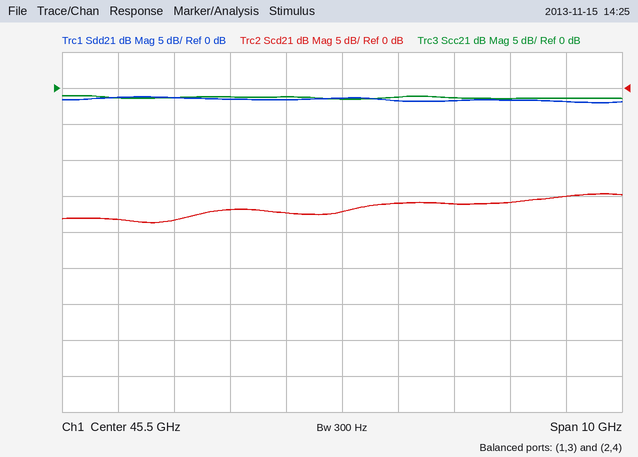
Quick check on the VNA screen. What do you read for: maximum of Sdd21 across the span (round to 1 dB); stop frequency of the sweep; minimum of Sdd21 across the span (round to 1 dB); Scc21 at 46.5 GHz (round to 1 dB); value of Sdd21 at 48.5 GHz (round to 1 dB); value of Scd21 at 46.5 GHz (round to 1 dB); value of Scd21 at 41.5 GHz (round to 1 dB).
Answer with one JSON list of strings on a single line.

["-1 dB", "50.5 GHz", "-2 dB", "-1 dB", "-2 dB", "-16 dB", "-18 dB"]
